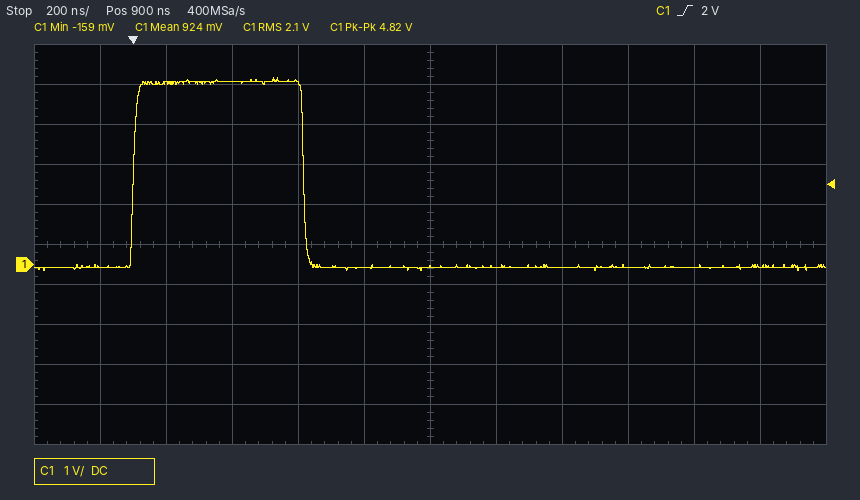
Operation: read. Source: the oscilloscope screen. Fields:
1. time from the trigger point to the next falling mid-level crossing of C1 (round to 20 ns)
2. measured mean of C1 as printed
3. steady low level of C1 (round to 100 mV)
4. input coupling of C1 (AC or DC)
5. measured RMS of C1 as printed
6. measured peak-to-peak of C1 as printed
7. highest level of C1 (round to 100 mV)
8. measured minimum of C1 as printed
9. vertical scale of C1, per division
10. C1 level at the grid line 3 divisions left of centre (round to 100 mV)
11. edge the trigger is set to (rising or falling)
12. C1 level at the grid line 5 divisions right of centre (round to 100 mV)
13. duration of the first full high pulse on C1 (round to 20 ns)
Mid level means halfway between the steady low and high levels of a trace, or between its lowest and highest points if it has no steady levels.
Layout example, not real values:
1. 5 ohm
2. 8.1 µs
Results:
1. 520 ns
2. 924 mV
3. -100 mV
4. DC
5. 2.1 V
6. 4.82 V
7. 4.7 V
8. -159 mV
9. 1 V
10. 4.6 V
11. rising
12. 0.0 V
13. 520 ns
